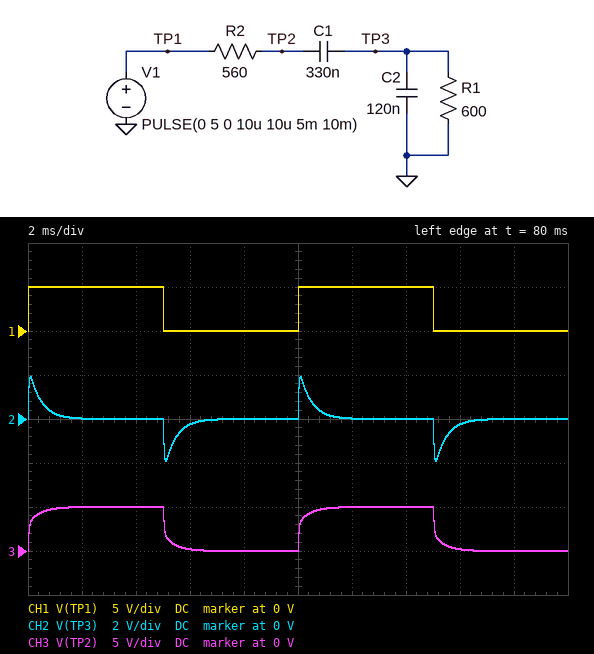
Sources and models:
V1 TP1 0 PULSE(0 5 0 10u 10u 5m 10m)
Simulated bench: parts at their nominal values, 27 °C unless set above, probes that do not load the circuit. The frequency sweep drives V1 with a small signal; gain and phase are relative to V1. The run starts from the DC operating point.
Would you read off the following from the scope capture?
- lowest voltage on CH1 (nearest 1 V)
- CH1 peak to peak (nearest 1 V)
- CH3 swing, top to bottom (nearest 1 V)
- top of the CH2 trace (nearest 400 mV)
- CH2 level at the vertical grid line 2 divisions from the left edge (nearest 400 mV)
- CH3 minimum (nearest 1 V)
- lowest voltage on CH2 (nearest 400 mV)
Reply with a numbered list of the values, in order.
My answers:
1. 0 V
2. 5 V
3. 5 V
4. 2.0 V
5. 0 V
6. 0 V
7. -2.0 V
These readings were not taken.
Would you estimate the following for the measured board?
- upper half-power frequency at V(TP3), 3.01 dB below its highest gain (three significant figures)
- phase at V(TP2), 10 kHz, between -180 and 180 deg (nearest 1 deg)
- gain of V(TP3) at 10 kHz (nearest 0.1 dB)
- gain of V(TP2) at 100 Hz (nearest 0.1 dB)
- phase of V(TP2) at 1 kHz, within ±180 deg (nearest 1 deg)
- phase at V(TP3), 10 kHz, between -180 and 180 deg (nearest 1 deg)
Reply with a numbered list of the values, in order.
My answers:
1. 5.77 kHz
2. -64 deg
3. -13.5 dB
4. -0.2 dB
5. -21 deg
6. -61 deg
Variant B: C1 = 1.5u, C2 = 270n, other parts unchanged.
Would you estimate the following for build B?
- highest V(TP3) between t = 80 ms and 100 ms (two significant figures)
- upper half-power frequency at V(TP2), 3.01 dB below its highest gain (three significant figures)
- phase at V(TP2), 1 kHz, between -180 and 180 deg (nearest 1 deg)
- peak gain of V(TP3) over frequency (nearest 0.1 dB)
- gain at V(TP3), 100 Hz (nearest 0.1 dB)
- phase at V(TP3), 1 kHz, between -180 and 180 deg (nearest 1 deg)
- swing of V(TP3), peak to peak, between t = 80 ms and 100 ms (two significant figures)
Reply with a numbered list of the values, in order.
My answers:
1. 2.0 V
2. 151 Hz
3. -29 deg
4. -6.5 dB
5. -8.6 dB
6. -20 deg
7. 4.0 V
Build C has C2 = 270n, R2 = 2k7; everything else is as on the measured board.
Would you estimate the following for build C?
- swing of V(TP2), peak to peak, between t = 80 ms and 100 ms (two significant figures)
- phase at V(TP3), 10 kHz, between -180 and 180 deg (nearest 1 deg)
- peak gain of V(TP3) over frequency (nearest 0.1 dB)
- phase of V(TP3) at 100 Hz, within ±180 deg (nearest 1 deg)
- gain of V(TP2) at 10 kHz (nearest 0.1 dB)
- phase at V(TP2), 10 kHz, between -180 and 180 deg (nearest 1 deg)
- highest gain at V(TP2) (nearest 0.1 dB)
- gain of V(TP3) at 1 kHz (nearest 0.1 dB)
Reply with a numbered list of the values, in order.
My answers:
1. 4.9 V
2. -82 deg
3. -16.0 dB
4. 50 deg
5. -28.1 dB
6. -85 deg
7. 0 dB
8. -17.3 dB
